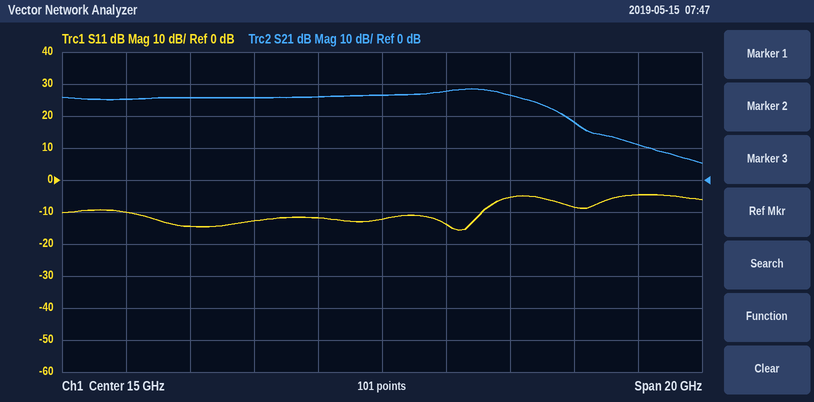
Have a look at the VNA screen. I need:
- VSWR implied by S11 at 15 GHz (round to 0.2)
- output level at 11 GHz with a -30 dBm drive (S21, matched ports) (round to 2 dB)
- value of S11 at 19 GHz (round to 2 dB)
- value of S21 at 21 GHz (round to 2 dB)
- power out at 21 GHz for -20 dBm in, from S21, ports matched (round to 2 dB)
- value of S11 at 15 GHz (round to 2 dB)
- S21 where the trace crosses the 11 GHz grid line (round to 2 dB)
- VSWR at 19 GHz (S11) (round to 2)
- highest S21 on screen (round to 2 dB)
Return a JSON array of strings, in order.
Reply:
["1.6", "-4 dBm", "-6 dB", "18 dB", "-2 dBm", "-12 dB", "26 dB", "4", "28 dB"]
